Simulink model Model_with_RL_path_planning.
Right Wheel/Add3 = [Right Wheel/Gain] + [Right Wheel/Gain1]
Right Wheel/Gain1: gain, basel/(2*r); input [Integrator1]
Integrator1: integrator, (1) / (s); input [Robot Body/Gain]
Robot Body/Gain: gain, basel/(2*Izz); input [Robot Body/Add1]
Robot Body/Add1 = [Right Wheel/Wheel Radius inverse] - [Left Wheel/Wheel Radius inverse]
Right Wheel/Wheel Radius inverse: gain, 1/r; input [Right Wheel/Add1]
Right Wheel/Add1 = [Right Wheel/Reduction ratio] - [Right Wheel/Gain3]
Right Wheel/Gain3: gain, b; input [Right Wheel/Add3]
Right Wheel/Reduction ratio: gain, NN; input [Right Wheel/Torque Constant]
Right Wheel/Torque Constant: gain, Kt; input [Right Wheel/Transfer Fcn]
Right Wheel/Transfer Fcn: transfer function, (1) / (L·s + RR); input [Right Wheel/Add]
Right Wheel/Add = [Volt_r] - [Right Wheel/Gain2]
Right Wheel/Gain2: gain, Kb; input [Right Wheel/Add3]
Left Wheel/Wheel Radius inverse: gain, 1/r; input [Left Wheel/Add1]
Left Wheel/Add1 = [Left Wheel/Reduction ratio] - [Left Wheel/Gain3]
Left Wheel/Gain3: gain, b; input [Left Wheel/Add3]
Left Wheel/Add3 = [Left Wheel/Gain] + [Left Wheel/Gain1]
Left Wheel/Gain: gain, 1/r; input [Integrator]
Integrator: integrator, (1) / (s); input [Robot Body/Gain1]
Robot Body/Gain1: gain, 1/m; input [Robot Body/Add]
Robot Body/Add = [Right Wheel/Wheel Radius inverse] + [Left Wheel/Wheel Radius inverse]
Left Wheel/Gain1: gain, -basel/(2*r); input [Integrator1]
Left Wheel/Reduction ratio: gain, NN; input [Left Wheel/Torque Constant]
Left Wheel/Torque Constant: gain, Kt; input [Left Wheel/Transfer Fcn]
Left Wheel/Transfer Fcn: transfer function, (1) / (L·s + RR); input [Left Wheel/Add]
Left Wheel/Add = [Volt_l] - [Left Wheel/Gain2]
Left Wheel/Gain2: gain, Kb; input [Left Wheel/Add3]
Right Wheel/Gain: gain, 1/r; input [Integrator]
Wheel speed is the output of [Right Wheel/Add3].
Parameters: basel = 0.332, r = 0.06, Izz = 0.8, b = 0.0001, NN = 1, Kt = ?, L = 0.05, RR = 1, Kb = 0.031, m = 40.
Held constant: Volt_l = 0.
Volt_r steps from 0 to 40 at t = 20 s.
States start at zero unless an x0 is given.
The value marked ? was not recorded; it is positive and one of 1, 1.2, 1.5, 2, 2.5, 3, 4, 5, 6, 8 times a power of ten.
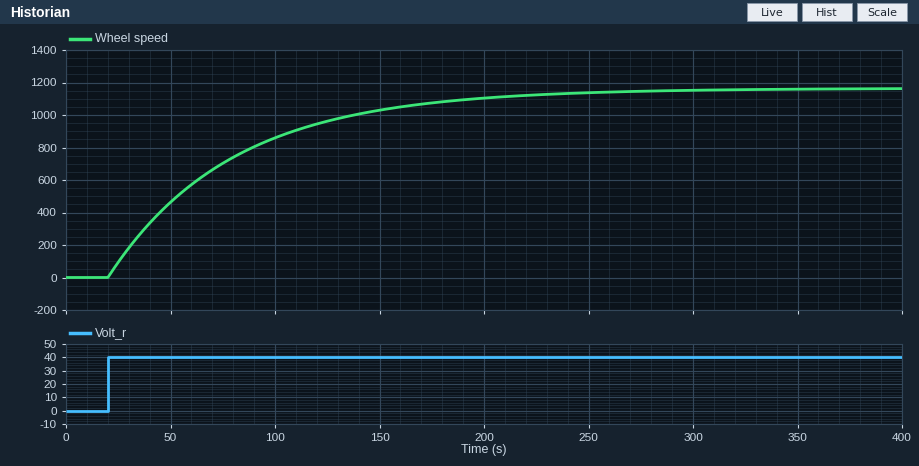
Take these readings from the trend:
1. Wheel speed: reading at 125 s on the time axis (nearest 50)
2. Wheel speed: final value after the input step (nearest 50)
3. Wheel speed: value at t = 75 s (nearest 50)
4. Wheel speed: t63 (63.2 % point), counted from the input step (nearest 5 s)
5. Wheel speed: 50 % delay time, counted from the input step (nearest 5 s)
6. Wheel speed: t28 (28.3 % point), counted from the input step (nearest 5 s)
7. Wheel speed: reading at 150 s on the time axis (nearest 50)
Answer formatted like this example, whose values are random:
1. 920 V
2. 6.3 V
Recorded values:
1. 950
2. 1150
3. 700
4. 60 s
5. 40 s
6. 20 s
7. 1050
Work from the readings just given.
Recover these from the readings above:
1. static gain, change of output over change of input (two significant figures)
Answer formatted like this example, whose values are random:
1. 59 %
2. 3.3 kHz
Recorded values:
1. 29
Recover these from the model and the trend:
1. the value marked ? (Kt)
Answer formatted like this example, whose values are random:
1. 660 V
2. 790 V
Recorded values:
1. 0.03
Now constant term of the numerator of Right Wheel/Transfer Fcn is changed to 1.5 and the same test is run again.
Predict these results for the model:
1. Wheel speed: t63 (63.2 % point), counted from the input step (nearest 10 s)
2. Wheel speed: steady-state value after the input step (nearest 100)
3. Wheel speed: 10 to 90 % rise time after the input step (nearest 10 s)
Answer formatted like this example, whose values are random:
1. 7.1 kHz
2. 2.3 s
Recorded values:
1. 40 s
2. 1200
3. 90 s
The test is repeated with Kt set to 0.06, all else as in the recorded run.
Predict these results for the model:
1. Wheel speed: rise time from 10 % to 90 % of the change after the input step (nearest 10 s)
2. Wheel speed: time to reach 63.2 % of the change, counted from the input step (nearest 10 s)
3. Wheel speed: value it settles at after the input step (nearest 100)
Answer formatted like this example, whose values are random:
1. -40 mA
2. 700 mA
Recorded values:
1. 70 s
2. 30 s
3. 1200
